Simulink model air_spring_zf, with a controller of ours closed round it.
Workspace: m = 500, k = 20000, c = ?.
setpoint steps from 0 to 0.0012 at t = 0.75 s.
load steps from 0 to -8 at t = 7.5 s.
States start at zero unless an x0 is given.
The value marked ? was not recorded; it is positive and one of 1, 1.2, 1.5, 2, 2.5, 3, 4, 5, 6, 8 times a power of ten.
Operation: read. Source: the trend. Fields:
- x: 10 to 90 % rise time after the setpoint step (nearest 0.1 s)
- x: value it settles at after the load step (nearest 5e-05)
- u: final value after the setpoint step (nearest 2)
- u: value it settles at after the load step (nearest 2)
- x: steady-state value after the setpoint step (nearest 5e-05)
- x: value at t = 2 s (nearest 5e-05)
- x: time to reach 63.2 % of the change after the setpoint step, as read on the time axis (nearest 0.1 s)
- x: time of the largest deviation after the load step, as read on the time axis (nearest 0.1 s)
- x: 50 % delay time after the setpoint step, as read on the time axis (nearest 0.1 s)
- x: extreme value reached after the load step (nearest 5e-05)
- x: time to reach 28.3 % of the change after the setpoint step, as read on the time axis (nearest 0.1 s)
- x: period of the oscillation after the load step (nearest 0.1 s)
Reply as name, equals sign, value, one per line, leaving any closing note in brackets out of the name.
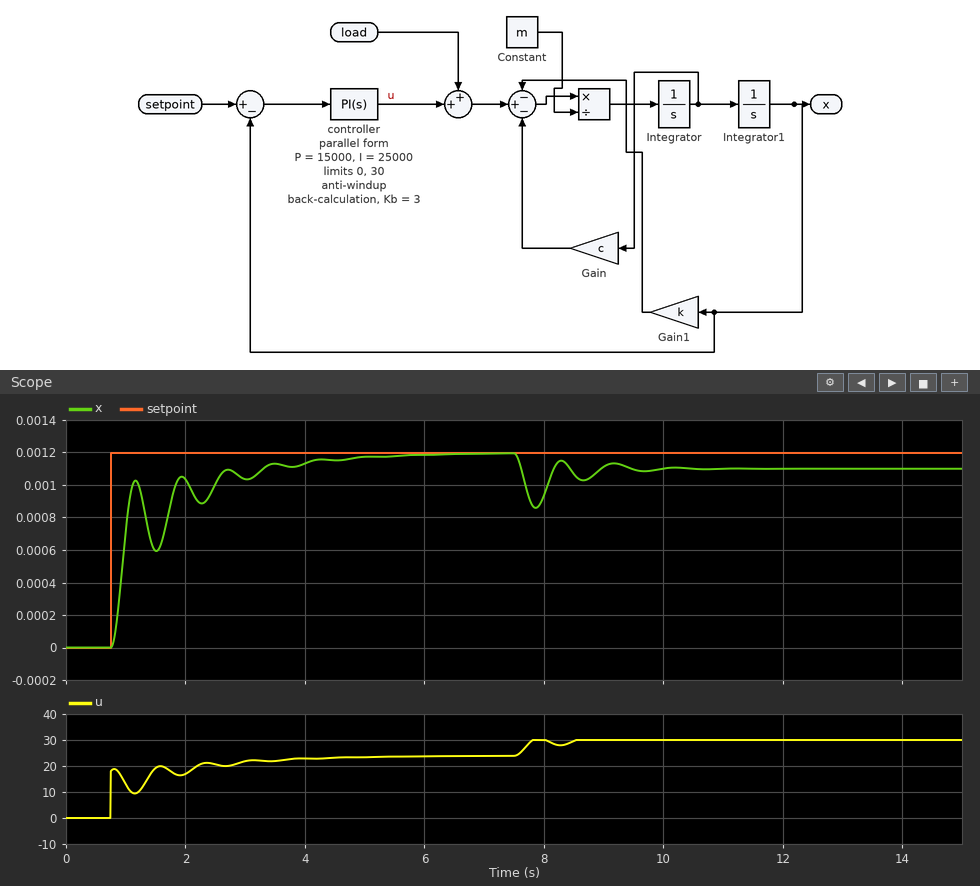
x: 10 to 90 % rise time after the setpoint step = 1.8 s
x: value it settles at after the load step = 0.00110
u: final value after the setpoint step = 24
u: value it settles at after the load step = 30
x: steady-state value after the setpoint step = 0.00120
x: value at t = 2 s = 0.00105
x: time to reach 63.2 % of the change after the setpoint step, as read on the time axis = 1.0 s
x: time of the largest deviation after the load step, as read on the time axis = 7.9 s
x: 50 % delay time after the setpoint step, as read on the time axis = 1.0 s
x: extreme value reached after the load step = 0.00085
x: time to reach 28.3 % of the change after the setpoint step, as read on the time axis = 0.9 s
x: period of the oscillation after the load step = 0.8 s
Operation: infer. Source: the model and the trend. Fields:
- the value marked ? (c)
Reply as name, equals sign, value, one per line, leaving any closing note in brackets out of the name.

the value marked ? = 1500
